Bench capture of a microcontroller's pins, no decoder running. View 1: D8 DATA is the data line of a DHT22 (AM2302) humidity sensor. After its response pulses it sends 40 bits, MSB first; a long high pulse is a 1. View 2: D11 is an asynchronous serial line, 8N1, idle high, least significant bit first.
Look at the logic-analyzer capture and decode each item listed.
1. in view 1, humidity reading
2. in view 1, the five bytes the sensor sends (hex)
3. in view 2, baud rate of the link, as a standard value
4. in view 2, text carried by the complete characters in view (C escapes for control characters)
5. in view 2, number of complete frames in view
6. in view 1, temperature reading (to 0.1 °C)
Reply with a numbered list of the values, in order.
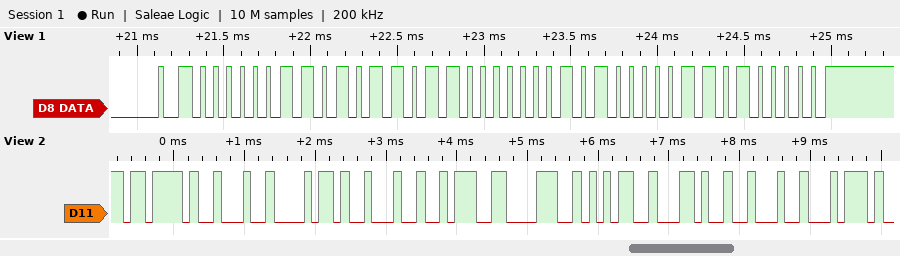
1. 85.9 %
2. 03 5B 01 41 A0
3. 9600 baud
4. "{\"h\":85,\"t"
5. 10
6. 32.1 °C
